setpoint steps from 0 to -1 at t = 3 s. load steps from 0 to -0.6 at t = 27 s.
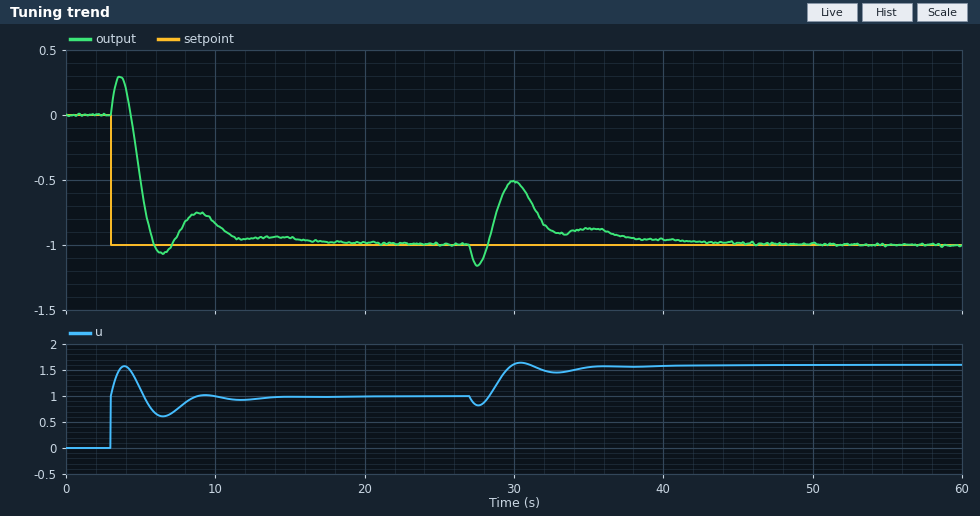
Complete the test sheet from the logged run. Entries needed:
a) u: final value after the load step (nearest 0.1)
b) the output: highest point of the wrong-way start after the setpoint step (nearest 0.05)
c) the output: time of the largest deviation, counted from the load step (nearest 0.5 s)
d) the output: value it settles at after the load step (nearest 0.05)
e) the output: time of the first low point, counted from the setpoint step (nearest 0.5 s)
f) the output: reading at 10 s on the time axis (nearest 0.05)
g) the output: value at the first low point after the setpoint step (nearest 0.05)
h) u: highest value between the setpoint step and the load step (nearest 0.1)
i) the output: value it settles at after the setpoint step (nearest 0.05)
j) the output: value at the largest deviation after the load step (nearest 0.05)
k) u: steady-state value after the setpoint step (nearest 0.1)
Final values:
1.6
0.30
3.0 s
-1.00
3.5 s
-0.85
-1.05
1.6
-1.00
-0.50
1.0
